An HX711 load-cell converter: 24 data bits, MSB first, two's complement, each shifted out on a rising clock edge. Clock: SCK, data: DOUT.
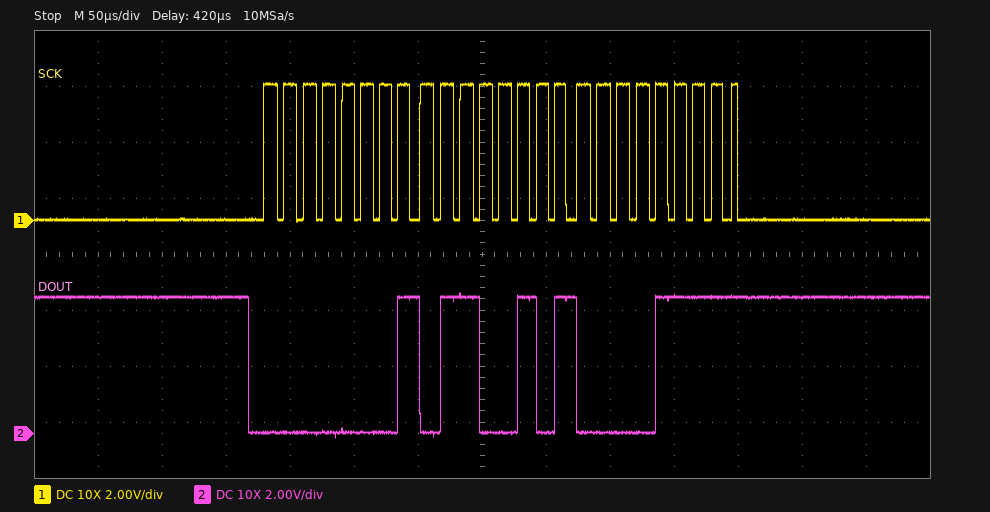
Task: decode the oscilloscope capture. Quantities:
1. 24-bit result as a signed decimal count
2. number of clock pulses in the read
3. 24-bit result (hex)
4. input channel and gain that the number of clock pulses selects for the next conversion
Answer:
91407
25
0x01650F
channel A, gain 128
